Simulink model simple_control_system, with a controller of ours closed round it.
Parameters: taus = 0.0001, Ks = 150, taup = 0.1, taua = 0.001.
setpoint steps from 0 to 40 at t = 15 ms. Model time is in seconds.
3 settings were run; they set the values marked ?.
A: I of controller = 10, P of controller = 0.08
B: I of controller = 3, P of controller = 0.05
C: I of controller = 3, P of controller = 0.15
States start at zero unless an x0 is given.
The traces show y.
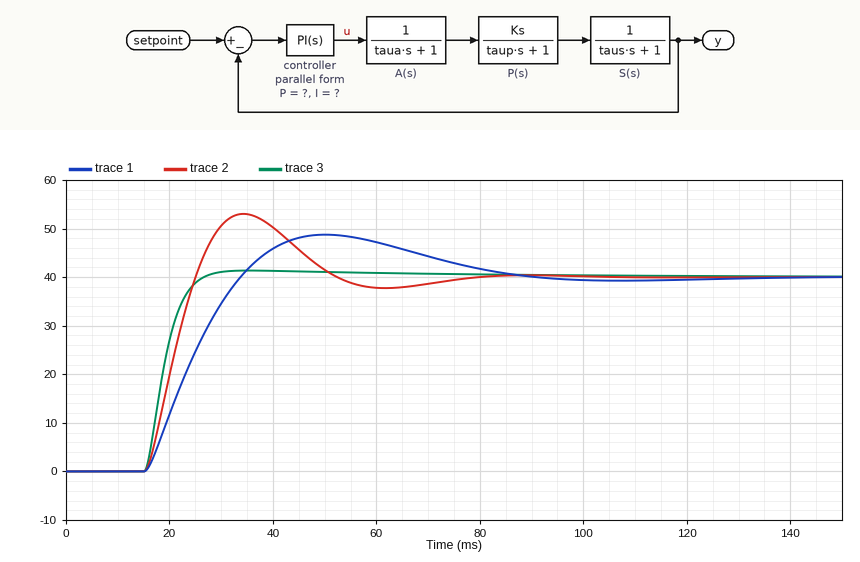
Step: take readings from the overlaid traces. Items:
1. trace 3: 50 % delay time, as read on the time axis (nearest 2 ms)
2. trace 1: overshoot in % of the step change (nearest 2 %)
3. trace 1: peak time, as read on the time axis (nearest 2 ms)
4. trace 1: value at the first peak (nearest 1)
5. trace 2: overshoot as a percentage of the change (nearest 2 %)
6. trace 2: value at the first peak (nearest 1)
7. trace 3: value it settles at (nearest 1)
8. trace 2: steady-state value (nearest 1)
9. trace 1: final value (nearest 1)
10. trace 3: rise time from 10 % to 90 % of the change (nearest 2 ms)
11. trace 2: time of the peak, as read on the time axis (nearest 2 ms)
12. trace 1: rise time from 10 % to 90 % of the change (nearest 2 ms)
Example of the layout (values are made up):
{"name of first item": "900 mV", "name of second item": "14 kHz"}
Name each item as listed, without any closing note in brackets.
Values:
{"trace 3: 50 % delay time, as read on the time axis": "18 ms", "trace 1: overshoot in % of the step change": "22 %", "trace 1: peak time, as read on the time axis": "50 ms", "trace 1: value at the first peak": "49", "trace 2: overshoot as a percentage of the change": "32 %", "trace 2: value at the first peak": "53", "trace 3: value it settles at": "40", "trace 2: steady-state value": "40", "trace 1: final value": "40", "trace 3: rise time from 10 % to 90 % of the change": "6 ms", "trace 2: time of the peak, as read on the time axis": "34 ms", "trace 1: rise time from 10 % to 90 % of the change": "14 ms"}
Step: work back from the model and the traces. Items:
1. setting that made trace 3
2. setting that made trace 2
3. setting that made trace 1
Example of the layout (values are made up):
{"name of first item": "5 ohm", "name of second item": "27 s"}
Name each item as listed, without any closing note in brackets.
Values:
{"setting that made trace 3": "C", "setting that made trace 2": "A", "setting that made trace 1": "B"}
